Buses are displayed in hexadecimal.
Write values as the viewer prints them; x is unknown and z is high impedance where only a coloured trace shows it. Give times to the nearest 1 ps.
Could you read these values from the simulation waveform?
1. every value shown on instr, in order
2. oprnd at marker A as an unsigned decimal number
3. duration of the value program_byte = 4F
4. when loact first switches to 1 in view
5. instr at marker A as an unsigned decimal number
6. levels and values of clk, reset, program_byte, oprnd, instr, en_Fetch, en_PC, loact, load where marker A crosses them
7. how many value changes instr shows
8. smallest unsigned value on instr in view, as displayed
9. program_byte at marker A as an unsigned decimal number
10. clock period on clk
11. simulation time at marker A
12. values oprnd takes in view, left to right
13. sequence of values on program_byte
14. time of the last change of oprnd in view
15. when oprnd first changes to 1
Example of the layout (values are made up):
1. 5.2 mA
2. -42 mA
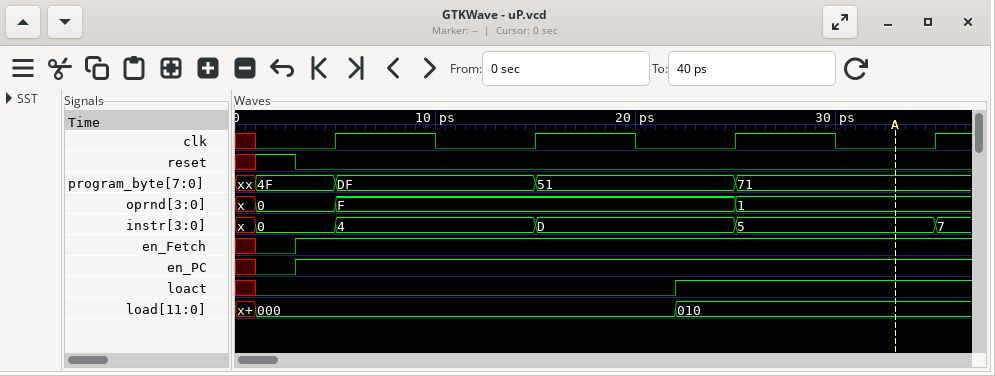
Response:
1. x, 0, 4, D, 5, 7
2. 1
3. 4 ps
4. 22 ps
5. 5
6. clk=0, reset=0, program_byte=71, oprnd=1, instr=5, en_Fetch=1, en_PC=1, loact=1, load=010
7. 5
8. 0
9. 113
10. 10 ps
11. 33 ps
12. x, 0, F, 1
13. xx, 4F, DF, 51, 71
14. 25 ps
15. 25 ps
